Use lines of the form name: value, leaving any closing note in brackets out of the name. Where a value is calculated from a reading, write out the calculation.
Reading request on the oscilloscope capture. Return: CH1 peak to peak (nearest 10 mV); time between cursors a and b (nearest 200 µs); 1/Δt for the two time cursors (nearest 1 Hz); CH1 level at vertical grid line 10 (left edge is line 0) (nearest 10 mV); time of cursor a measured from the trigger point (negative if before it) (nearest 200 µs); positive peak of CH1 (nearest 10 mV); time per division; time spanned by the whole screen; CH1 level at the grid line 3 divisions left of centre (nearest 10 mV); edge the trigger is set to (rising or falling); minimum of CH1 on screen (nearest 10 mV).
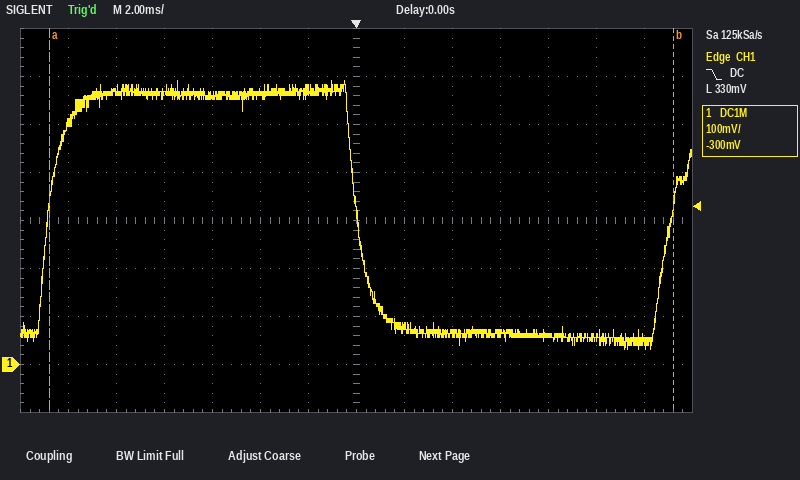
CH1 peak to peak: 590 mV − (30 mV) = 560 mV
time between cursors a and b: 26.0 ms
1/Δt for the two time cursors: 1 / 26.0 ms ≈ 38 Hz
CH1 level at vertical grid line 10 (left edge is line 0): 60 mV
time of cursor a measured from the trigger point (negative if before it): -12.8 ms
positive peak of CH1: 590 mV
time per division: 2 ms
time spanned by the whole screen: 28 ms
CH1 level at the grid line 3 divisions left of centre: 560 mV
edge the trigger is set to: falling
minimum of CH1 on screen: 30 mV
